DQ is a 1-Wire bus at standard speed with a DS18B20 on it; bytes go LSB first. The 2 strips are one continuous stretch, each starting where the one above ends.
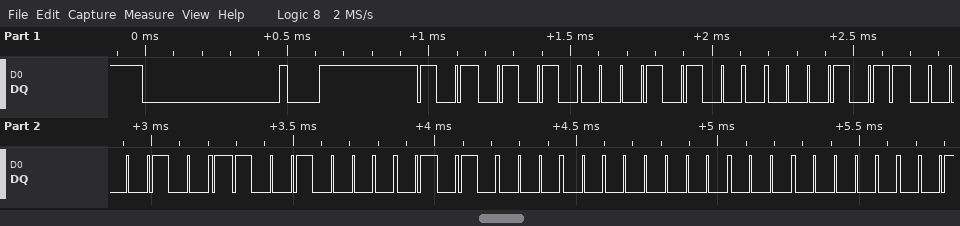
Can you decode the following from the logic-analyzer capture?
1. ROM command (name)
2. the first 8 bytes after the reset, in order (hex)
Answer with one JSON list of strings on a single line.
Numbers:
["Match ROM", "55 28 D0 90 09 0A 00 00"]
